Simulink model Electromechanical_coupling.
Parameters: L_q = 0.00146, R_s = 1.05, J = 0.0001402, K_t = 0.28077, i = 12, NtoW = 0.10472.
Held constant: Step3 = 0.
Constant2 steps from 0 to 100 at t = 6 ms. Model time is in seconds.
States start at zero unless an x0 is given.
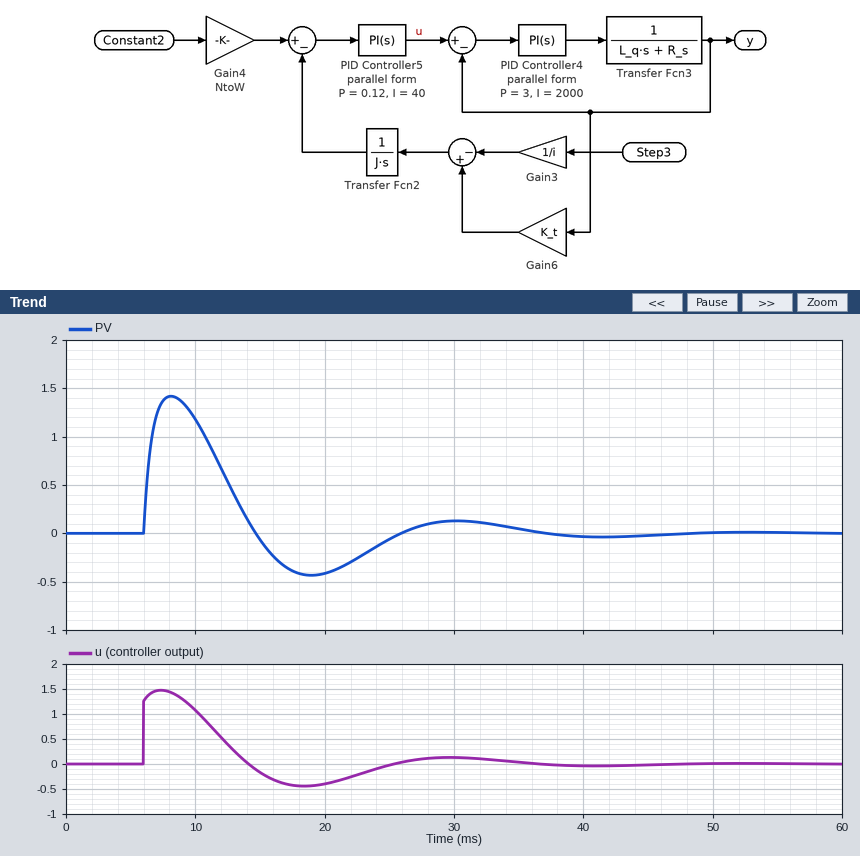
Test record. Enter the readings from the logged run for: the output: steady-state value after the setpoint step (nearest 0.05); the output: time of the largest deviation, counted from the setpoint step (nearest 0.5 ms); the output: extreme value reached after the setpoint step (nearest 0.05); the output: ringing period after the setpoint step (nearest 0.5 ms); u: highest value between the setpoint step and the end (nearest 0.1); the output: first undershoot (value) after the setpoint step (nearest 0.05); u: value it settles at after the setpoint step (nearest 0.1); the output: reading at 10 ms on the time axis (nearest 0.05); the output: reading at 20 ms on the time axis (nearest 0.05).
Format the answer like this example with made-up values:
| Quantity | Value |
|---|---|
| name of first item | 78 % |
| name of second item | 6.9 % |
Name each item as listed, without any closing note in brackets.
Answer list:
| Quantity | Value |
|---|---|
| the output: steady-state value after the setpoint step | 0.00 |
| the output: time of the largest deviation, counted from the setpoint step | 2.0 ms |
| the output: extreme value reached after the setpoint step | 1.40 |
| the output: ringing period after the setpoint step | 22.0 ms |
| u: highest value between the setpoint step and the end | 1.5 |
| the output: first undershoot (value) after the setpoint step | -0.45 |
| u: value it settles at after the setpoint step | 0.0 |
| the output: reading at 10 ms on the time axis | 1.20 |
| the output: reading at 20 ms on the time axis | -0.40 |
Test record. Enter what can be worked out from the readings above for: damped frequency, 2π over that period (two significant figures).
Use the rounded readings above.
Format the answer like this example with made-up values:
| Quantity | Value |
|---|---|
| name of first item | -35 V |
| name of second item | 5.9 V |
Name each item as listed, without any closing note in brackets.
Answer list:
| Quantity | Value |
|---|---|
| damped frequency, 2π over that period | 0.29 rad/ms |
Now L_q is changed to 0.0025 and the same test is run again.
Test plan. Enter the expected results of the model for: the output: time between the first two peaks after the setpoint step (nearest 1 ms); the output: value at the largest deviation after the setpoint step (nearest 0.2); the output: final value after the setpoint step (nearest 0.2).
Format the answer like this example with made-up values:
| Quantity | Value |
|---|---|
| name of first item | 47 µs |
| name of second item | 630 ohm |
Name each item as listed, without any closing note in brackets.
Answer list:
| Quantity | Value |
|---|---|
| the output: time between the first two peaks after the setpoint step | 21 ms |
| the output: value at the largest deviation after the setpoint step | 1.6 |
| the output: final value after the setpoint step | 0.0 |
